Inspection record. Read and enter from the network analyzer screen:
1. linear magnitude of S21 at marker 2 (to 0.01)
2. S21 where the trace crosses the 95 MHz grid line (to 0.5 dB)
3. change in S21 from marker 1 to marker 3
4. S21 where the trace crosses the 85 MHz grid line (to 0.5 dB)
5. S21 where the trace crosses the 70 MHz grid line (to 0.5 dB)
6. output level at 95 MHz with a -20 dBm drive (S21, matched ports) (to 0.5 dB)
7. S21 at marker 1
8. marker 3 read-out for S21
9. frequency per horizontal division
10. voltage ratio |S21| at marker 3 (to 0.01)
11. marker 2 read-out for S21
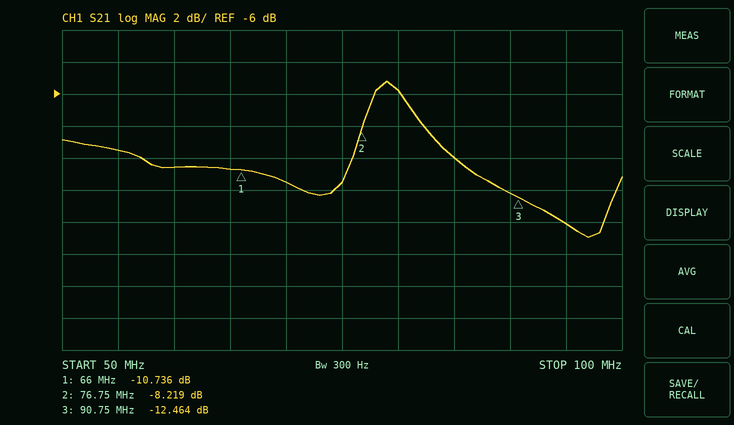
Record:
0.39
-14.0 dB
-1.728 dB
-10.0 dB
-11.5 dB
-34.0 dBm
-10.736 dB
-12.464 dB
5 MHz
0.24
-8.219 dB
